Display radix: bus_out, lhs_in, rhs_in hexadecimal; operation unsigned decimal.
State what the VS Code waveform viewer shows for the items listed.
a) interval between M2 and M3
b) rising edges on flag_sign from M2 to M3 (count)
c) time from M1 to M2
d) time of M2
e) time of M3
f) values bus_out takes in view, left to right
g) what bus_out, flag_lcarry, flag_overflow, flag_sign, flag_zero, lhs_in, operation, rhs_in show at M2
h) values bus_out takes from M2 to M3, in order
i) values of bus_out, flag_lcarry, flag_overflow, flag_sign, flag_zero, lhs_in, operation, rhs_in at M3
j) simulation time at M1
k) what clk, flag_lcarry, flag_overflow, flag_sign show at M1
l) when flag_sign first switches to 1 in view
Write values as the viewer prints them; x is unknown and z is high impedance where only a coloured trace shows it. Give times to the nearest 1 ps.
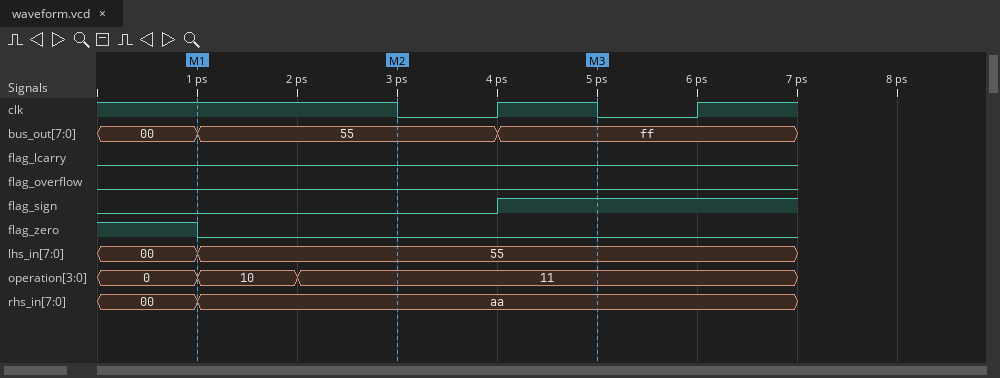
2 ps
1
2 ps
3 ps
5 ps
00, 55, ff
bus_out=55, flag_lcarry=0, flag_overflow=0, flag_sign=0, flag_zero=0, lhs_in=55, operation=11, rhs_in=aa
55, ff
bus_out=ff, flag_lcarry=0, flag_overflow=0, flag_sign=1, flag_zero=0, lhs_in=55, operation=11, rhs_in=aa
1 ps
clk=1, flag_lcarry=0, flag_overflow=0, flag_sign=0
4 ps
